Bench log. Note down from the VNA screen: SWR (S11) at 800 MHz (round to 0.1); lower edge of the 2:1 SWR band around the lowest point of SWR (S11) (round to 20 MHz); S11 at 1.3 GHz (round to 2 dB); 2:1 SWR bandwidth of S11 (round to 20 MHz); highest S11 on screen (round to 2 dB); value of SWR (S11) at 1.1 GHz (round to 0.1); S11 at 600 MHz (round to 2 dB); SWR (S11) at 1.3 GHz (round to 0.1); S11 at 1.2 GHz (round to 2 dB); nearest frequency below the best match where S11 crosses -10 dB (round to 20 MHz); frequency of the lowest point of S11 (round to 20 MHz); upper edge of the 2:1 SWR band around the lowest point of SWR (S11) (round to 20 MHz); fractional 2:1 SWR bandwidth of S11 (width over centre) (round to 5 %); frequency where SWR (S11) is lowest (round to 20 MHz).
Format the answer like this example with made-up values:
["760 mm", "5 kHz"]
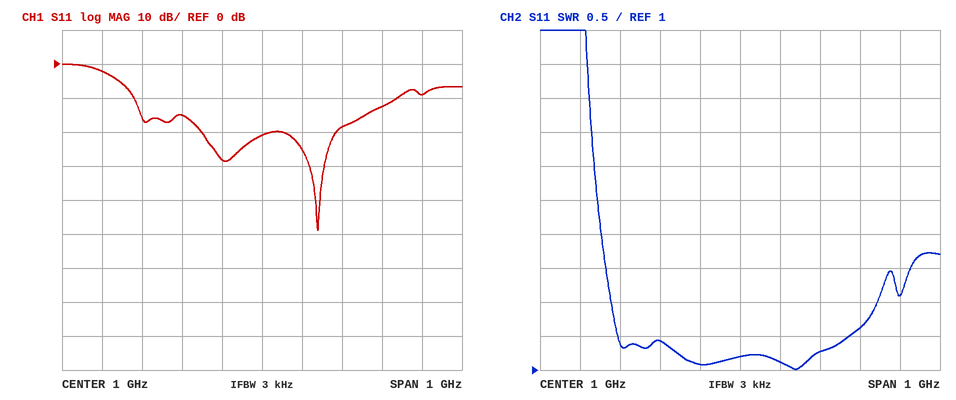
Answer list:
["1.4", "680 MHz", "-12 dB", "660 MHz", "0 dB", "1.1", "-2 dB", "1.6", "-18 dB", "680 MHz", "1.14 GHz", "1.34 GHz", "65 %", "1.14 GHz"]
